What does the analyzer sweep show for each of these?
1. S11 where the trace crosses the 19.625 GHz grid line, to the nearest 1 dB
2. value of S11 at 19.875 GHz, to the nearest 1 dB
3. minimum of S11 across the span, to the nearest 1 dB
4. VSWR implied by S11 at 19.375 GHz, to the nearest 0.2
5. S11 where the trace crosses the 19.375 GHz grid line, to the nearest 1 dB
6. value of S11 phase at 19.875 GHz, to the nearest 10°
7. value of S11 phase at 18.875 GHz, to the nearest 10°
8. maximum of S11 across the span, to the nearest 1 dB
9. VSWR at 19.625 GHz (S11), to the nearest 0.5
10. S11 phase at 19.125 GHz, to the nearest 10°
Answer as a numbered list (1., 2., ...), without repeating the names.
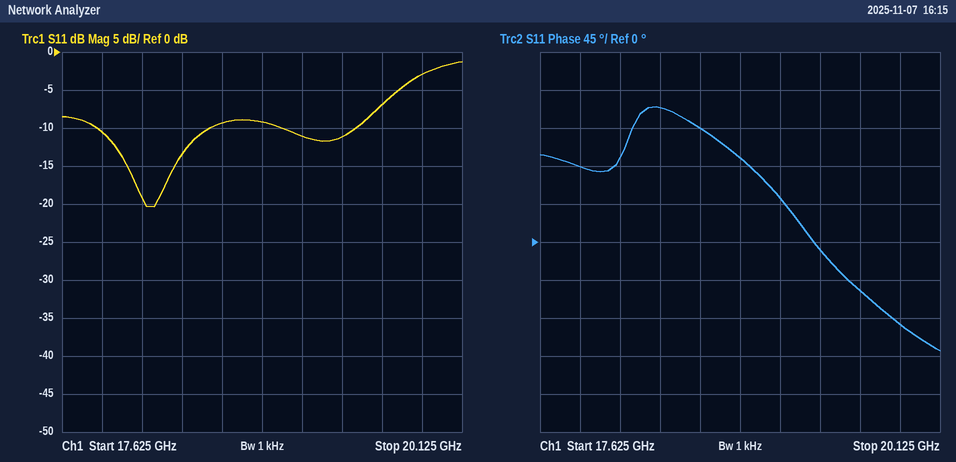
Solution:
1. -7 dB
2. -3 dB
3. -20 dB
4. 1.8
5. -11 dB
6. -100°
7. 100°
8. -1 dB
9. 2.5
10. 50°
